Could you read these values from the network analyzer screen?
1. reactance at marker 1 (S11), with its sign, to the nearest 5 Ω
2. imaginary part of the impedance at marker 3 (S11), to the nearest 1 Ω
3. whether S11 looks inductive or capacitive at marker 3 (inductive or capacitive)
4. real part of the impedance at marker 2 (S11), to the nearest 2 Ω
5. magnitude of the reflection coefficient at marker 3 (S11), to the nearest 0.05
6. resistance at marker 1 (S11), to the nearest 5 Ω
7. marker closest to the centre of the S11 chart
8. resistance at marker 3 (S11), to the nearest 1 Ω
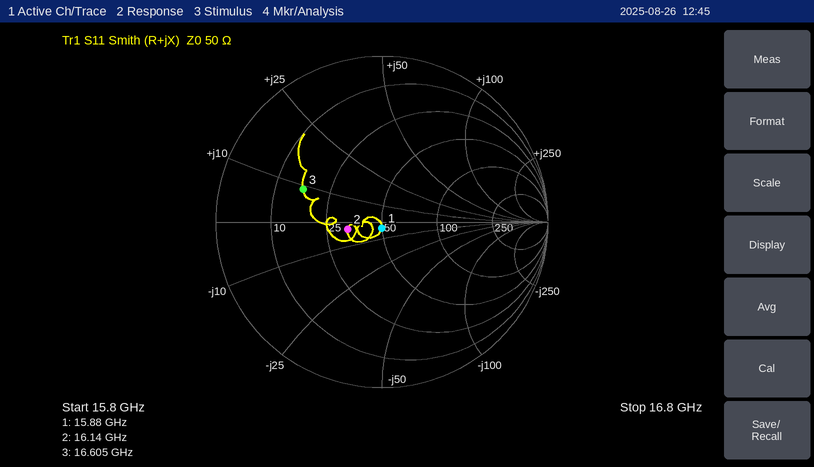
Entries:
-5 Ω
+9 Ω
inductive
32 Ω
0.50
50 Ω
marker 1
17 Ω
